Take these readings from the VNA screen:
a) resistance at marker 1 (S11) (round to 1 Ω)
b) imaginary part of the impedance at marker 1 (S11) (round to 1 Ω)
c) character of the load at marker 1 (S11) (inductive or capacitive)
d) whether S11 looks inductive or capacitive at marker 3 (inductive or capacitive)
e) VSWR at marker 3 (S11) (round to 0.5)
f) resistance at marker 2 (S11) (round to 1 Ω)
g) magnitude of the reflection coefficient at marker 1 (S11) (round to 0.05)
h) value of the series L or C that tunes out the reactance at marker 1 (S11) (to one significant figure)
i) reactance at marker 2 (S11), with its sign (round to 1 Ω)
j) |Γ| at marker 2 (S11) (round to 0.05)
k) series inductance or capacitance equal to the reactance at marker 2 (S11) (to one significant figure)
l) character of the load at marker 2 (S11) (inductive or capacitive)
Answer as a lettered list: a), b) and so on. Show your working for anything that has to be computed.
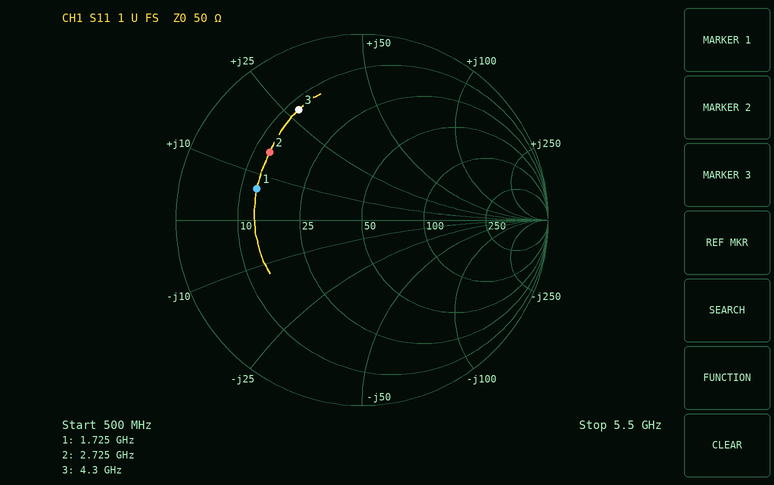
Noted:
a) 13 Ω
b) +7 Ω
c) inductive
d) inductive
e) 5.5
f) 13 Ω
g) 0.60
h) C = 1/(2π × 1.725 GHz × 7 Ω) ≈ 13.2 pF, so 10 pF to one significant figure
i) +15 Ω
j) 0.60
k) L = 15 Ω/(2π × 2.725 GHz) ≈ 876 pH, so 900 pH to one significant figure
l) inductive
